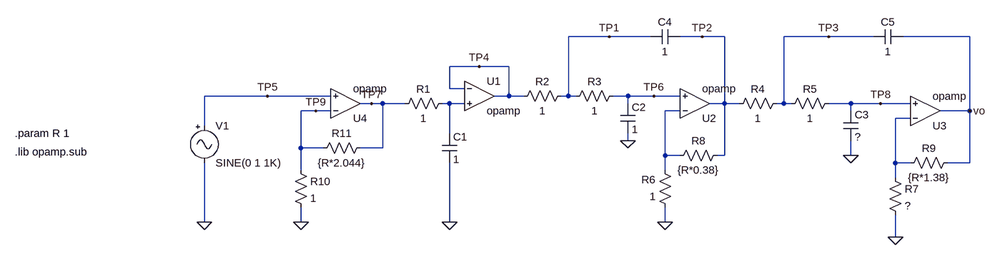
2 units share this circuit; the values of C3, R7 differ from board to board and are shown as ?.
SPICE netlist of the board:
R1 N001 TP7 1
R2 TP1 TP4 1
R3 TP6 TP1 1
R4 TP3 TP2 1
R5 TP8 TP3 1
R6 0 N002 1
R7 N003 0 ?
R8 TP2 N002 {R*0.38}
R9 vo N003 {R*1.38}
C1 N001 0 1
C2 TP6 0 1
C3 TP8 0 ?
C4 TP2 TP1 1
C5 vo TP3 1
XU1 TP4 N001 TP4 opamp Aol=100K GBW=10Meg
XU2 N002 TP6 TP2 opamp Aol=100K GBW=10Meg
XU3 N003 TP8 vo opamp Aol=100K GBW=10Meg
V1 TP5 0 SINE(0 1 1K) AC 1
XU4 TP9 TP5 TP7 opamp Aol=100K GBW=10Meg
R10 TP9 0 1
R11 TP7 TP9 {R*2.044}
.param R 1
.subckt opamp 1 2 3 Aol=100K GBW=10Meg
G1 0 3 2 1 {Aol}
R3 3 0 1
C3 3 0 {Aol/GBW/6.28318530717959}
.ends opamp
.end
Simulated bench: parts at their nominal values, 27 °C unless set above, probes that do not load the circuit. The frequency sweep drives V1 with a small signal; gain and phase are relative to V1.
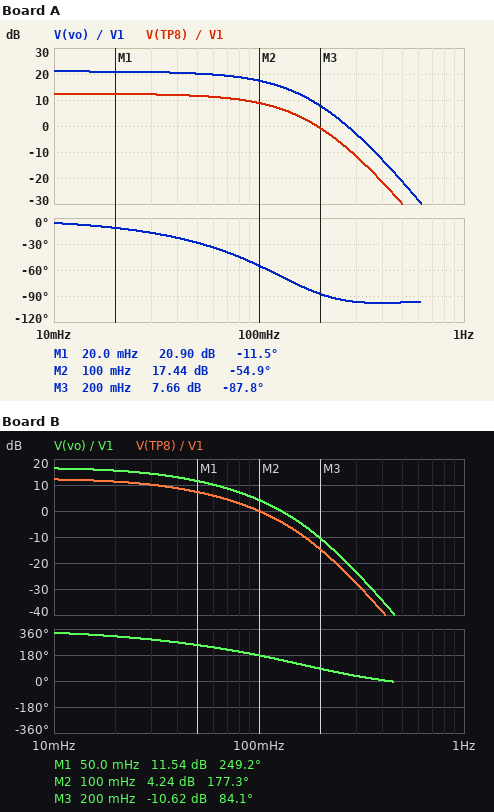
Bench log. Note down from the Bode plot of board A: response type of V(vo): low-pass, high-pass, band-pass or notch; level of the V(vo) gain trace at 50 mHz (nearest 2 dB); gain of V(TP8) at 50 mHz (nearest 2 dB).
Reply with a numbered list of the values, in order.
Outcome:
1. low-pass
2. 20 dB
3. 12 dB
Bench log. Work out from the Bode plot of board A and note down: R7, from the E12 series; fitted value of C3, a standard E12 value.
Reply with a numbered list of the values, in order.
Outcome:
1. 0.82 Ω
2. 330 mF
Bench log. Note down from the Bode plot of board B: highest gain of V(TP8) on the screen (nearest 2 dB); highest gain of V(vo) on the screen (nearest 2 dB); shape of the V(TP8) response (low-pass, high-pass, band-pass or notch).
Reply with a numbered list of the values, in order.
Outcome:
1. 12 dB
2. 16 dB
3. low-pass
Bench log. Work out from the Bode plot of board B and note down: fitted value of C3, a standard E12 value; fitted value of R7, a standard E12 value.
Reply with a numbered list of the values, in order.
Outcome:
1. 2.7 F
2. 2.2 Ω
